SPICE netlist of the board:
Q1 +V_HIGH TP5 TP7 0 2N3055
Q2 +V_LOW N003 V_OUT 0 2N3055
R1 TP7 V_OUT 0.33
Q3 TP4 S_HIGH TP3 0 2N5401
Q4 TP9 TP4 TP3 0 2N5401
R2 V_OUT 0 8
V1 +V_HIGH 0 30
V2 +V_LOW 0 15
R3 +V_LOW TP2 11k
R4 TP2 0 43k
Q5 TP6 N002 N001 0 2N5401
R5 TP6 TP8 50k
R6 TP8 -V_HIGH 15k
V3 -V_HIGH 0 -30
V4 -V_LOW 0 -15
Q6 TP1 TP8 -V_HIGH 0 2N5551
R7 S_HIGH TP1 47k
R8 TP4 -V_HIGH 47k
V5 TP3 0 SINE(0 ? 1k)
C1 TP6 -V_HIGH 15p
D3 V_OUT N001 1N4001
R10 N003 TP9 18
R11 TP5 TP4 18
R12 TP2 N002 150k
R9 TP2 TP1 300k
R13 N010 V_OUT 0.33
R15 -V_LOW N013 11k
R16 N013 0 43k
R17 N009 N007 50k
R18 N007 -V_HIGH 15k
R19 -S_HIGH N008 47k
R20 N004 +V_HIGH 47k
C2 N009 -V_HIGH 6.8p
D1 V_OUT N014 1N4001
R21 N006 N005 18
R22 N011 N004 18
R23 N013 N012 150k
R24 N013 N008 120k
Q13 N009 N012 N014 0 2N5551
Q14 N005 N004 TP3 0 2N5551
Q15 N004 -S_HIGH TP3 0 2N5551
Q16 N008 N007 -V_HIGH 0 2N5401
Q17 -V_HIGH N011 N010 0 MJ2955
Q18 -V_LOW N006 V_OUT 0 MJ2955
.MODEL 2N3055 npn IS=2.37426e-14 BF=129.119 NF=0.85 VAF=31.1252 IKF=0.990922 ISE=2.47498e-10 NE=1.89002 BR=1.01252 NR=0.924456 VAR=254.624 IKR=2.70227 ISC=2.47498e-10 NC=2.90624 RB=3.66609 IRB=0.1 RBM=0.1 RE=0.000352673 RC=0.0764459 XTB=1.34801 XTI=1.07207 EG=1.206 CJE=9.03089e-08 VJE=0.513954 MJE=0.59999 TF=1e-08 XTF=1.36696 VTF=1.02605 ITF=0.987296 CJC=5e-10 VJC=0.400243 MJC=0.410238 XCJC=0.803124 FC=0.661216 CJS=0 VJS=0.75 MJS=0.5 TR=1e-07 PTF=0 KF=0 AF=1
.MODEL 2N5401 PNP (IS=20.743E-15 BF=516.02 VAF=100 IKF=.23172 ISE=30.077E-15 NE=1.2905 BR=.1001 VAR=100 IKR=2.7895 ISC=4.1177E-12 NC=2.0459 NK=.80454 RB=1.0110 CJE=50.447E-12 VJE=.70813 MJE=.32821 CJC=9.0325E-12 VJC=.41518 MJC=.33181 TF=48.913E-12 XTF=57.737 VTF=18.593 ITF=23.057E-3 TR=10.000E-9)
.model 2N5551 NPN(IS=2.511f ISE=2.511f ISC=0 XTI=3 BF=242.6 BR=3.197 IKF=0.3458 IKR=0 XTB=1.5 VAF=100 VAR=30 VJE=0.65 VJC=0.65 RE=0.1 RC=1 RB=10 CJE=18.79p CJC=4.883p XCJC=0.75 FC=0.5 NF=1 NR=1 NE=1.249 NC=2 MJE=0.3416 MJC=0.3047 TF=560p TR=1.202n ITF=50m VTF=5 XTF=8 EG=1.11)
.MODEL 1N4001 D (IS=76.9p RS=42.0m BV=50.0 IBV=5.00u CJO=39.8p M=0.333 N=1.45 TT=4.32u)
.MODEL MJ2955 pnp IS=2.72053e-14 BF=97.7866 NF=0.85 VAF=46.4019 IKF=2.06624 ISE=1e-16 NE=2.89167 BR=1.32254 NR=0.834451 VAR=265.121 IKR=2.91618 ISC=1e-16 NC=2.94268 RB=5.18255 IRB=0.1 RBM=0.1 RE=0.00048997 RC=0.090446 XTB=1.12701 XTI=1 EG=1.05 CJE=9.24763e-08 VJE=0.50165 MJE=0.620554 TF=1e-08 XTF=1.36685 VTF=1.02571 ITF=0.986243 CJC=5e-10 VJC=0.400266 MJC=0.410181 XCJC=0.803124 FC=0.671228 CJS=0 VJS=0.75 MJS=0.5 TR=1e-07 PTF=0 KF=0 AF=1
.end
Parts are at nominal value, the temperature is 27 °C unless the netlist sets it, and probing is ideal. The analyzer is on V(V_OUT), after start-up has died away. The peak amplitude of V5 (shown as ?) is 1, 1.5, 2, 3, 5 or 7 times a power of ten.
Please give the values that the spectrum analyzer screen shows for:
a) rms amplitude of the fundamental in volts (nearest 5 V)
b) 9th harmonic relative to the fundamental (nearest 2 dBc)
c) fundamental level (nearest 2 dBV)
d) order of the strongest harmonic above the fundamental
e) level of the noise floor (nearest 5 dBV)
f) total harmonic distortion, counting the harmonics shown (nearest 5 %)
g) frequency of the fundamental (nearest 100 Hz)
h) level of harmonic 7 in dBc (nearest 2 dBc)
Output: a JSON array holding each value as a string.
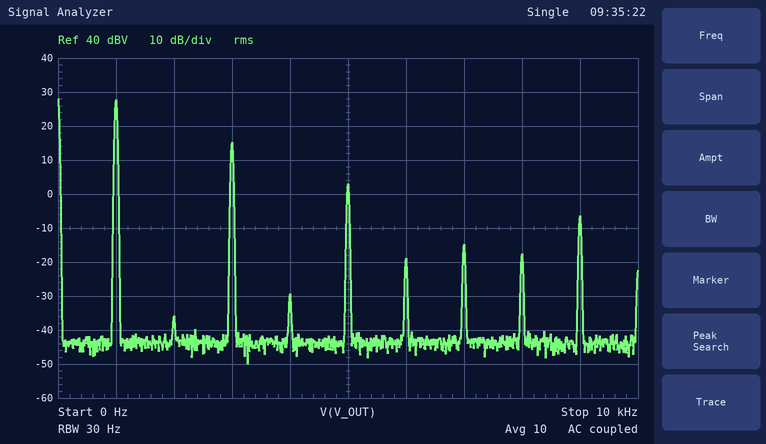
["25 V", "-34 dBc", "28 dBV", "3", "-45 dBV", "25 %", "1.0 kHz", "-42 dBc"]
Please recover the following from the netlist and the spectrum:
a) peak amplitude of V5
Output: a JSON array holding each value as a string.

["70 V"]
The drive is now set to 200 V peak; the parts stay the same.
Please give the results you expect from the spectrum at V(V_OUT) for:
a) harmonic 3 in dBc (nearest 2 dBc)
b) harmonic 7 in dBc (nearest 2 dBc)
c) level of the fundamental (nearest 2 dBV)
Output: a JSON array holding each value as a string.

["-10 dBc", "-18 dBc", "28 dBV"]
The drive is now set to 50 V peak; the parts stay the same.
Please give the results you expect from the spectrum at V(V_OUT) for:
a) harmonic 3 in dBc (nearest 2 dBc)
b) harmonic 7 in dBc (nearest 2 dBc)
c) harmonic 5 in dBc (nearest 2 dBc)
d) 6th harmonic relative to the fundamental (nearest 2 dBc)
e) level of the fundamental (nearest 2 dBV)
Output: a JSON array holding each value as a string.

["-16 dBc", "-34 dBc", "-38 dBc", "-42 dBc", "28 dBV"]
